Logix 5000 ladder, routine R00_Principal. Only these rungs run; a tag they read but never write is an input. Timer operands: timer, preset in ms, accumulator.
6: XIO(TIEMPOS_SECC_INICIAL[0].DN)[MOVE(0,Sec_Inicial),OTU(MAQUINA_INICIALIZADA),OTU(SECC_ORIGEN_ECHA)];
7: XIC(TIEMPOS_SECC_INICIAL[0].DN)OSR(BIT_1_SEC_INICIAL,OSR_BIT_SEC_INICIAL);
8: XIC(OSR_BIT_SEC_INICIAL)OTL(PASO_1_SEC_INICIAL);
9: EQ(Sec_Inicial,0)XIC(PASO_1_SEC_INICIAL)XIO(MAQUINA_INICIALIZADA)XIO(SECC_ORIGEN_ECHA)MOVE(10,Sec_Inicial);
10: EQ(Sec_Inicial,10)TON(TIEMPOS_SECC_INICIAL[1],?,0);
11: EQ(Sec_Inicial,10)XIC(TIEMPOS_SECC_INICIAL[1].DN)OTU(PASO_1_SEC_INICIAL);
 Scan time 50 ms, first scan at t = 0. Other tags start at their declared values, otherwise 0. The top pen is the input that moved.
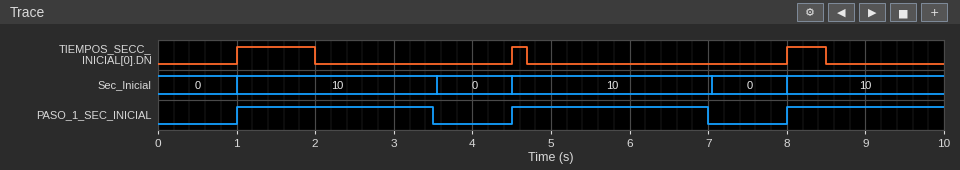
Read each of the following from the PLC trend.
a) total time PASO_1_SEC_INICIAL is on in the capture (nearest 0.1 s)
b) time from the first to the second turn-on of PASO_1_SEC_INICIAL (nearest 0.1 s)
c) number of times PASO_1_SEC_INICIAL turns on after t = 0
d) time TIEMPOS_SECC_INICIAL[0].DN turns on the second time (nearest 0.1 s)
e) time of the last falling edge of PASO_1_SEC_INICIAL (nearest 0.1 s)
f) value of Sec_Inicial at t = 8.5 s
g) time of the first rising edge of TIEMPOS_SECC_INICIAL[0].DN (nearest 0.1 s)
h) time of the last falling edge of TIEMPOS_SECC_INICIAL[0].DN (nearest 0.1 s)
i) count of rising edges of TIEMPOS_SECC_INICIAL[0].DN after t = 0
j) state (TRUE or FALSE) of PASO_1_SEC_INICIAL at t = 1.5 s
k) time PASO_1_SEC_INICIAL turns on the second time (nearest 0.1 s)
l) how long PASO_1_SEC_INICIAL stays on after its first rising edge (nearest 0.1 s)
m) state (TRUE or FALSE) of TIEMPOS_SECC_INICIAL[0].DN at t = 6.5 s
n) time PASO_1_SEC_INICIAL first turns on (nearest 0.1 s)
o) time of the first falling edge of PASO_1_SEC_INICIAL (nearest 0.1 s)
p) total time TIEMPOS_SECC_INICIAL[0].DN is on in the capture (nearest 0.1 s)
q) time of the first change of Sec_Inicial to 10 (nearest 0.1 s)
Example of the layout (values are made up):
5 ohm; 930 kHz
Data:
7.0 s; 3.5 s; 3; 4.5 s; 7.0 s; 10; 1.0 s; 8.5 s; 3; TRUE; 4.5 s; 2.5 s; FALSE; 1.0 s; 3.5 s; 1.7 s; 1.0 s
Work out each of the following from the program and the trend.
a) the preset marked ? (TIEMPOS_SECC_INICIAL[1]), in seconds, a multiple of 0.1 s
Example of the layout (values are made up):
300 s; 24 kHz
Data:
2.5 s
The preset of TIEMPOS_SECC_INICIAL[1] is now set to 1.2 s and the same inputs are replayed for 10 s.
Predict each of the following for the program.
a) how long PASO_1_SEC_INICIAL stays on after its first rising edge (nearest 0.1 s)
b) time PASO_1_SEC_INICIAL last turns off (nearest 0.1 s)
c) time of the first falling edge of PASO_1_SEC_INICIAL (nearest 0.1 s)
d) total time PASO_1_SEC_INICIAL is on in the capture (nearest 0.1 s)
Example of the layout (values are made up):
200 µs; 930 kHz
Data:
1.2 s; 9.2 s; 2.2 s; 3.6 s
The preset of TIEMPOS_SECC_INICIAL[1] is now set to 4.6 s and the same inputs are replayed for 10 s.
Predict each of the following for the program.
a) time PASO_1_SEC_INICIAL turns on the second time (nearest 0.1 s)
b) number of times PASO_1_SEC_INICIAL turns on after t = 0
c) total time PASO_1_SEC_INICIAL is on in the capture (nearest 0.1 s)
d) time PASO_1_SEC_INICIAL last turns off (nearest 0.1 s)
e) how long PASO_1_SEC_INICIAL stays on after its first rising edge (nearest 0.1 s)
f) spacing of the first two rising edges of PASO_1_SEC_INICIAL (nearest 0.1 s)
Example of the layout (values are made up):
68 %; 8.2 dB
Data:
8.0 s; 2; 6.6 s; 5.6 s; 4.6 s; 7.0 s
